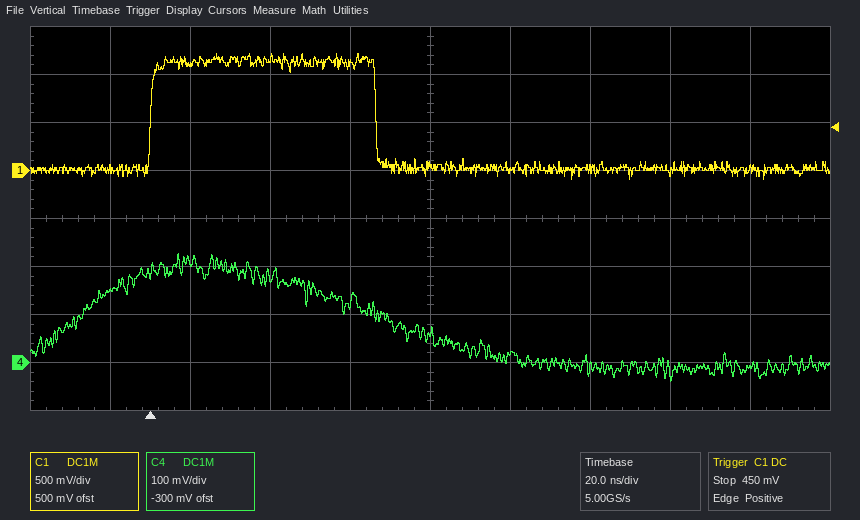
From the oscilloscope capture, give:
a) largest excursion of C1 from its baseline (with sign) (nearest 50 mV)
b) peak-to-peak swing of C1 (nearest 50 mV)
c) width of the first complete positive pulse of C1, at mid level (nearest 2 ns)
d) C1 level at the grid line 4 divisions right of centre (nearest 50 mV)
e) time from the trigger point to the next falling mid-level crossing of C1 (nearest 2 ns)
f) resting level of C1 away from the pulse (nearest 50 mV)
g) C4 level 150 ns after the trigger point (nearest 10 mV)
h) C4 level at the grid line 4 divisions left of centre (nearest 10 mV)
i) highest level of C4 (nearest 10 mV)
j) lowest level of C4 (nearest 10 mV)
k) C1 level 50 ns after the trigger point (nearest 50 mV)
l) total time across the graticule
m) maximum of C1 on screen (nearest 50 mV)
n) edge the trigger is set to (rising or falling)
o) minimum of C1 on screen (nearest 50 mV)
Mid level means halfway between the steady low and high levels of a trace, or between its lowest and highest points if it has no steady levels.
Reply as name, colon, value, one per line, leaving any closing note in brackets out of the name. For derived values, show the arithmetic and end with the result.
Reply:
largest excursion of C1 from its baseline (with sign): 1.20 V − (0 mV) = +1.20 V
peak-to-peak swing of C1: 1.20 V − (-100 mV) = 1.30 V
width of the first complete positive pulse of C1, at mid level: 56 ns
C1 level at the grid line 4 divisions right of centre: 0 mV
time from the trigger point to the next falling mid-level crossing of C1: 56 ns
resting level of C1 away from the pulse: 0 mV
C4 level 150 ns after the trigger point: -10 mV
C4 level at the grid line 4 divisions left of centre: 150 mV
highest level of C4: 230 mV
lowest level of C4: -40 mV
C1 level 50 ns after the trigger point: 1.10 V
total time across the graticule: 200 ns
maximum of C1 on screen: 1.20 V
edge the trigger is set to: rising
minimum of C1 on screen: -100 mV
